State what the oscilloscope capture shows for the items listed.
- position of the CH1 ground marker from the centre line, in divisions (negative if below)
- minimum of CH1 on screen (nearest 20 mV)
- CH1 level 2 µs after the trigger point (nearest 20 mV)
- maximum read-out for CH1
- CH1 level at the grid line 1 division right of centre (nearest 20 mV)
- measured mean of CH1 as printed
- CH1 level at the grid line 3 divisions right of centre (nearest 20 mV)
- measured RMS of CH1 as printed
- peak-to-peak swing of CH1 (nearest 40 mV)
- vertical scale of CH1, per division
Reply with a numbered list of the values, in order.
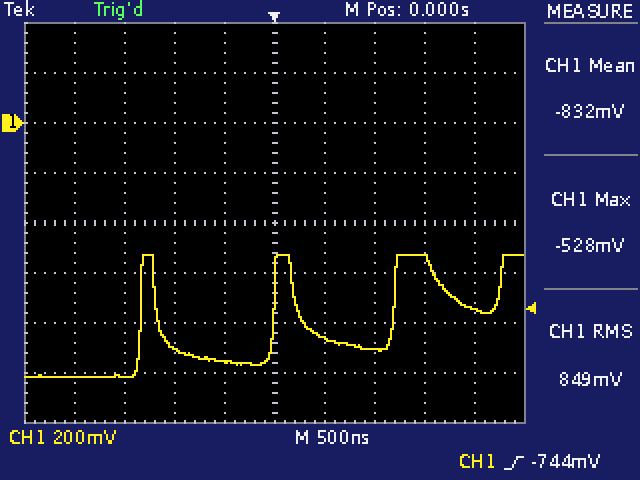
1. +2.0 div
2. -1.02 V
3. -740 mV
4. -528 mV
5. -860 mV
6. -832 mV
7. -540 mV
8. 849 mV
9. 480 mV
10. 200 mV
